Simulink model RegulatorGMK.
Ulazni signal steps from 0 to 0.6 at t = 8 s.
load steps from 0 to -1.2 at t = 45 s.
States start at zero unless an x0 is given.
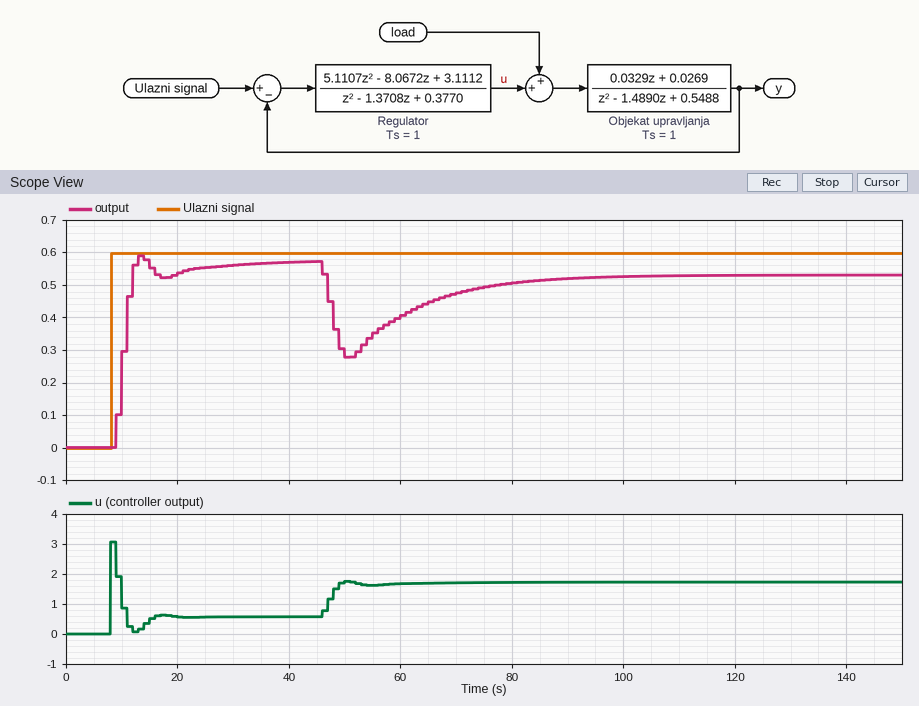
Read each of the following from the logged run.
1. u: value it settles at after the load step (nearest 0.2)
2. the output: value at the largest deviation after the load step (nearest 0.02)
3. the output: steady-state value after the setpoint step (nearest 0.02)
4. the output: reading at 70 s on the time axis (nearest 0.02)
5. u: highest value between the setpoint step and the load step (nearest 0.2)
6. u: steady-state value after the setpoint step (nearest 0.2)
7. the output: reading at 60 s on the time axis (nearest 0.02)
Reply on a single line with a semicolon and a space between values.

1.8; 0.28; 0.58; 0.48; 3.0; 0.6; 0.40
